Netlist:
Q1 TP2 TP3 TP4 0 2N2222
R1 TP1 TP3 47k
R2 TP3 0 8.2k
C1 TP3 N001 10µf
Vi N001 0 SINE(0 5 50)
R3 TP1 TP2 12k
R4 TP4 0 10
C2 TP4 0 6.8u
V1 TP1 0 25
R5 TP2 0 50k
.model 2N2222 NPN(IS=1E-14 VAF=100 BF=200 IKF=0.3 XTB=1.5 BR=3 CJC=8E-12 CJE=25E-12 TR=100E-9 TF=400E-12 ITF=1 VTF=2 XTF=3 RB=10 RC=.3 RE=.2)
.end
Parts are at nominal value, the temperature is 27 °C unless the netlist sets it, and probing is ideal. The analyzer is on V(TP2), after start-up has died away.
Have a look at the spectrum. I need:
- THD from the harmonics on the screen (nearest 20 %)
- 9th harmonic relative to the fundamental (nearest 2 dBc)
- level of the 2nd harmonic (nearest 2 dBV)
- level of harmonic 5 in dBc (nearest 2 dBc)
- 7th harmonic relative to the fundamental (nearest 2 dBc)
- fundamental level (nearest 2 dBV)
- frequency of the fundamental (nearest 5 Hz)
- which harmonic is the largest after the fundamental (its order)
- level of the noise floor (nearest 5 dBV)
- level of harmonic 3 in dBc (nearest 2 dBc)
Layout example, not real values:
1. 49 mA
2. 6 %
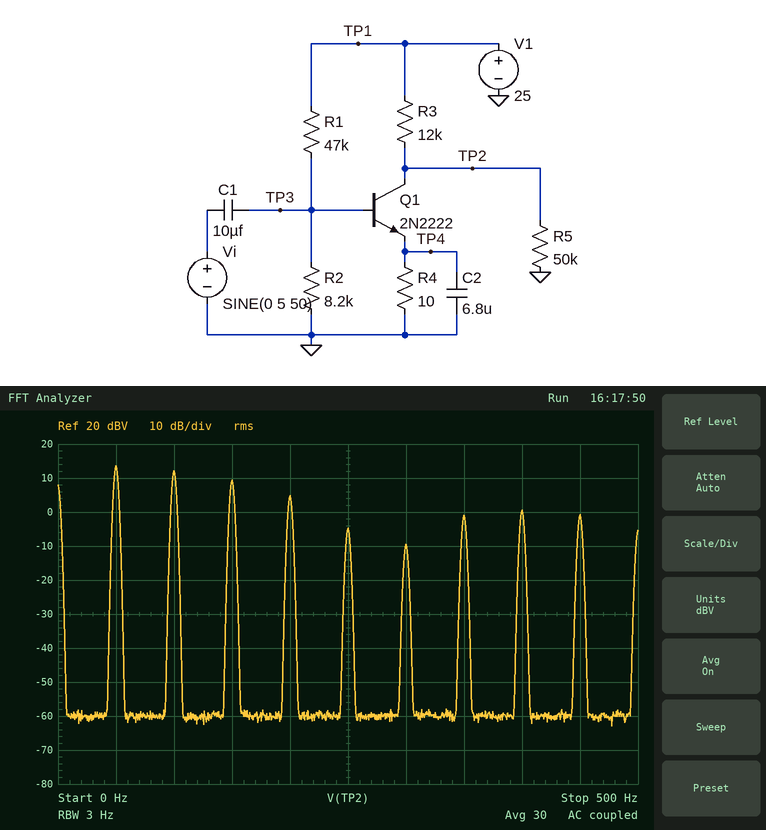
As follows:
1. 120 %
2. -14 dBc
3. 12 dBV
4. -18 dBc
5. -14 dBc
6. 14 dBV
7. 50 Hz
8. 2
9. -60 dBV
10. -4 dBc
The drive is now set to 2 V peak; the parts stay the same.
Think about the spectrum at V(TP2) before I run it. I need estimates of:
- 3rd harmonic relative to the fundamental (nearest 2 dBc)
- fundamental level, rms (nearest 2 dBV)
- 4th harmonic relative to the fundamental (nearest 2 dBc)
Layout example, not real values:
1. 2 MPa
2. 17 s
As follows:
1. -8 dBc
2. 16 dBV
3. -22 dBc
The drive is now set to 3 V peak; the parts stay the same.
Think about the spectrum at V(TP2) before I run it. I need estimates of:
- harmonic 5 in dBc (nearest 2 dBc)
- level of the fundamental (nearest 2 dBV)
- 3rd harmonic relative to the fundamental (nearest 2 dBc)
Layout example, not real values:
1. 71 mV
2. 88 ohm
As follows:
1. -34 dBc
2. 14 dBV
3. -6 dBc
